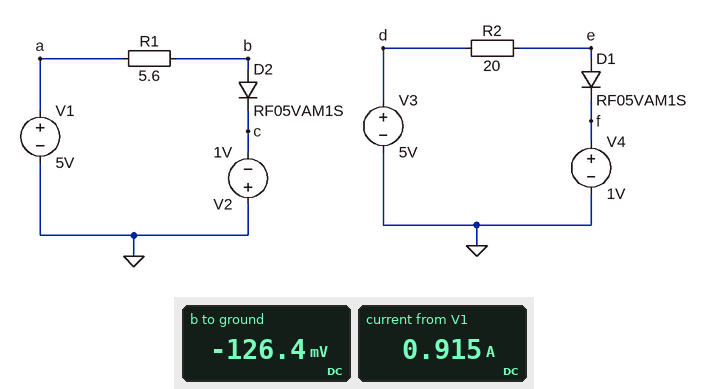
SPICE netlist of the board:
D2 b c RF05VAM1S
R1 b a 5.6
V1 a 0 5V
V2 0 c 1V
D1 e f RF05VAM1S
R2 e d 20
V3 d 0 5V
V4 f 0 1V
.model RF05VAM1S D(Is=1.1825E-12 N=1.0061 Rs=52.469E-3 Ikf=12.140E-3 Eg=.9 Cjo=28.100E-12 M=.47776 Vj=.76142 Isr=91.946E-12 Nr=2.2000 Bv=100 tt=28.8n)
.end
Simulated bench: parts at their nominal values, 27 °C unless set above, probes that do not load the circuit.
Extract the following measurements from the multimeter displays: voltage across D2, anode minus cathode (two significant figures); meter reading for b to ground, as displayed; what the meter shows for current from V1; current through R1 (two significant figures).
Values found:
870 mV
-126.4 mV
0.915 A
920 mA
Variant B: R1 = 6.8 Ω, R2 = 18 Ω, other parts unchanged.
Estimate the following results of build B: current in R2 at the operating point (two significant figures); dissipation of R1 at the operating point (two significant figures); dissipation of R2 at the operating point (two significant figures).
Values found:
180 mA
3.9 W
590 mW
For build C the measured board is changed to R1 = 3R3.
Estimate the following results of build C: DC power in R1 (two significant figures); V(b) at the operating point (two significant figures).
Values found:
7.8 W
-67 mV
